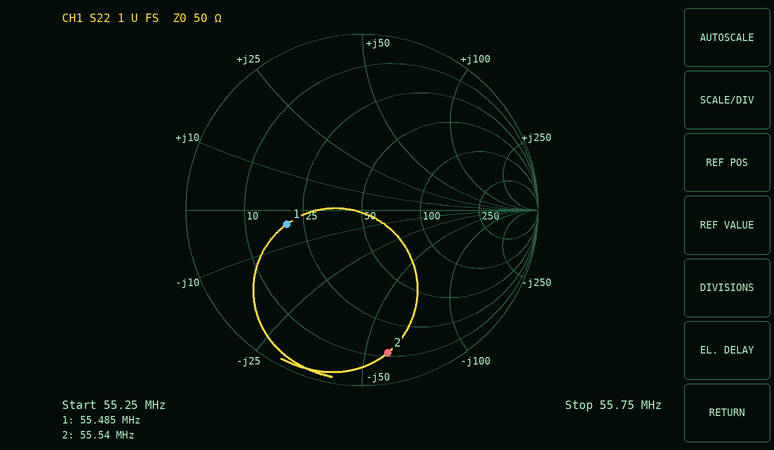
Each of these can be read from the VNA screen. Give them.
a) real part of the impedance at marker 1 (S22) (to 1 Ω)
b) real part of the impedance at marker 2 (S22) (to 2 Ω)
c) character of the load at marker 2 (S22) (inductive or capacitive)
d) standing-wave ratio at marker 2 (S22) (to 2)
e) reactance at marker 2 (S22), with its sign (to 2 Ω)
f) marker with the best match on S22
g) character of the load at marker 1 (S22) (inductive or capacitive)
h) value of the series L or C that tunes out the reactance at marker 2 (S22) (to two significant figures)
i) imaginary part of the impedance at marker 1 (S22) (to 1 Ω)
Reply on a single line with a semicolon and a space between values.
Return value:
20 Ω; 12 Ω; capacitive; 10; -58 Ω; marker 1; capacitive; 170 nH; -4 Ω
